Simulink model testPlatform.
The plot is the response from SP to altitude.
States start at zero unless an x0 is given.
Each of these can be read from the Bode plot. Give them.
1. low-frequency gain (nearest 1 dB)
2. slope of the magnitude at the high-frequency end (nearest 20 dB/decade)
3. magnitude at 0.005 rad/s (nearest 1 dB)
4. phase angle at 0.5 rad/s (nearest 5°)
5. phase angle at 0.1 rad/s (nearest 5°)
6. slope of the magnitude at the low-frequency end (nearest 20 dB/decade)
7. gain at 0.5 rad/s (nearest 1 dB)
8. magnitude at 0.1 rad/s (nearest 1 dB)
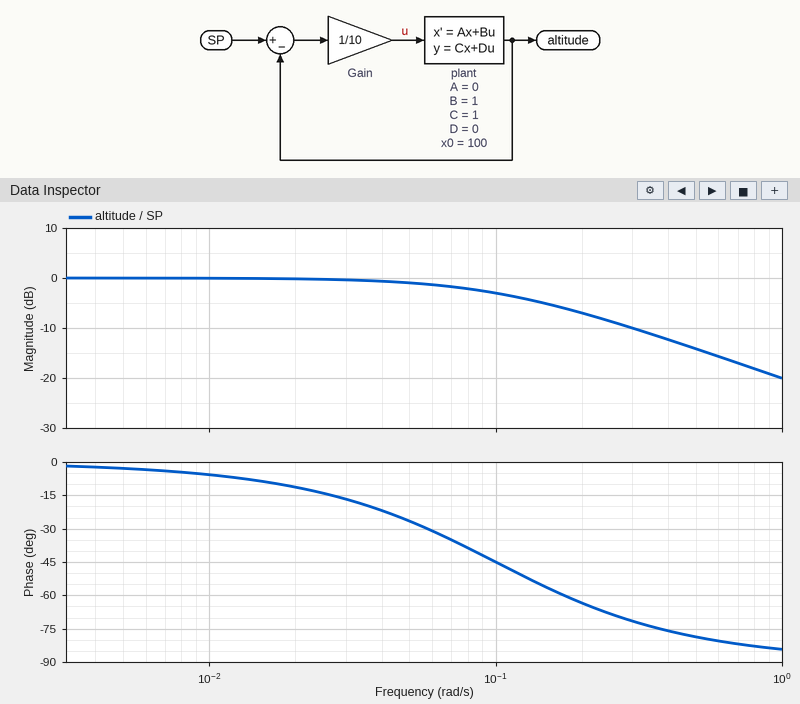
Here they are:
0 dB
-20 dB/decade
0 dB
-80°
-45°
0 dB/decade
-14 dB
-3 dB
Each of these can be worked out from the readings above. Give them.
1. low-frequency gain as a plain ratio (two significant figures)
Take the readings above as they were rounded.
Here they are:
1.0
